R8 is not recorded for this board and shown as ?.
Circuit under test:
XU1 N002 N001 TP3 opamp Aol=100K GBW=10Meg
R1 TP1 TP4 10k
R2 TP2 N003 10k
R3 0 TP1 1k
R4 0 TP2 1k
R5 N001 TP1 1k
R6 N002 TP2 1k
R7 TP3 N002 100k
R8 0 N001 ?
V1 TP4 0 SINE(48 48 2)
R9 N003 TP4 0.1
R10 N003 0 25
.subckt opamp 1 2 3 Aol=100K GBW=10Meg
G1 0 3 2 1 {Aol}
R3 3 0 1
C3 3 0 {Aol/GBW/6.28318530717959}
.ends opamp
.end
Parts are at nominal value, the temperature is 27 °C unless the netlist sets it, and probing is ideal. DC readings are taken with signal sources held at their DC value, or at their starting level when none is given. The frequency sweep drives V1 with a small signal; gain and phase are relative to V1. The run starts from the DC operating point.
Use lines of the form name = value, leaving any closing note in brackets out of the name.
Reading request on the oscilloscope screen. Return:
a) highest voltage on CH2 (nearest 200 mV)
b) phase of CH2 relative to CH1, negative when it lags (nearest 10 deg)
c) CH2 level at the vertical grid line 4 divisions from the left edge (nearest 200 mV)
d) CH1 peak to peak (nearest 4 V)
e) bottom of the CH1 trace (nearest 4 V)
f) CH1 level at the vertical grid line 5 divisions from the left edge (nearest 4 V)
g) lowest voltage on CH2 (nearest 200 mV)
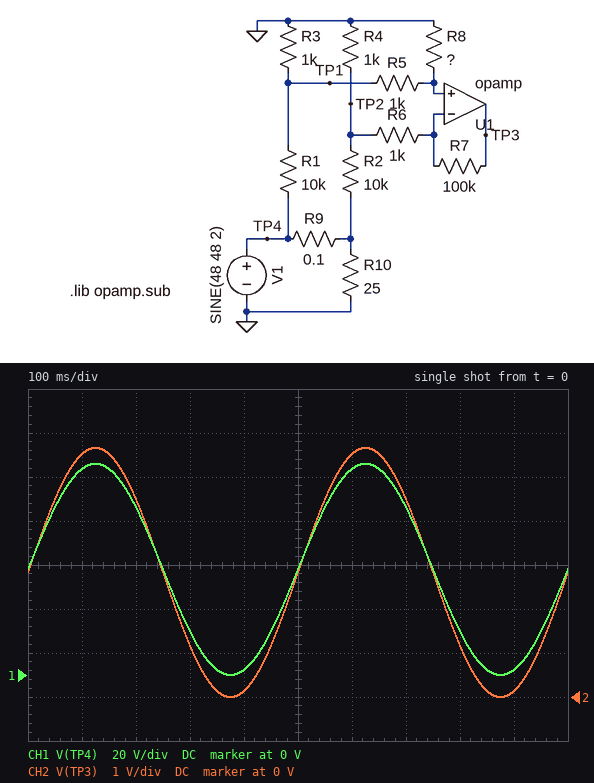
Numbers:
highest voltage on CH2 = 5.6 V
phase of CH2 relative to CH1, negative when it lags = 0 deg
CH2 level at the vertical grid line 4 divisions from the left edge = 200 mV
CH1 peak to peak = 96 V
bottom of the CH1 trace = 0 V
CH1 level at the vertical grid line 5 divisions from the left edge = 48 V
lowest voltage on CH2 = 0 V
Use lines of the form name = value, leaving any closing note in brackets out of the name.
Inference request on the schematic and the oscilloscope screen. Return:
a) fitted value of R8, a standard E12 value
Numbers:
fitted value of R8, a standard E12 value = 180 kΩ
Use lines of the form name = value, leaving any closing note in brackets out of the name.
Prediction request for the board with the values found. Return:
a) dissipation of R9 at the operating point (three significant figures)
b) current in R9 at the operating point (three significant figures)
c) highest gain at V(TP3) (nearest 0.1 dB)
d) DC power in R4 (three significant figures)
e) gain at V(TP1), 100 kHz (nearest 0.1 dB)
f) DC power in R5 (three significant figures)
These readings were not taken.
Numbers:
dissipation of R9 at the operating point = 367 mW
current in R9 at the operating point = 1.92 A
highest gain at V(TP3) = -24.6 dB
DC power in R4 = 18.8 mW
gain at V(TP1), 100 kHz = -20.9 dB
DC power in R5 = 575 nW
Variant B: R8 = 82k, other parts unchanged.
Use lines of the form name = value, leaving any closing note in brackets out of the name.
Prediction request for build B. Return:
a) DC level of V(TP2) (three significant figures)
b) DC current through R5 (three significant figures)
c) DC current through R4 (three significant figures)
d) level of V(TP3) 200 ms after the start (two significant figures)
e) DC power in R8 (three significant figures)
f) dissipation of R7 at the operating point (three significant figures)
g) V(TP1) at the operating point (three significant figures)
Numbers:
DC level of V(TP2) = 4.31 V
DC current through R5 = 52.0 µA
DC current through R4 = 4.31 mA
level of V(TP3) 200 ms after the start = -37 mV
DC power in R8 = 222 µW
dissipation of R7 at the operating point = 184 µW
V(TP1) at the operating point = 4.32 V
